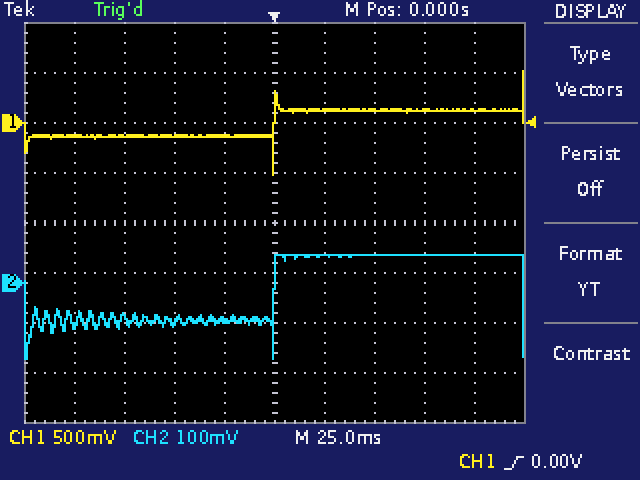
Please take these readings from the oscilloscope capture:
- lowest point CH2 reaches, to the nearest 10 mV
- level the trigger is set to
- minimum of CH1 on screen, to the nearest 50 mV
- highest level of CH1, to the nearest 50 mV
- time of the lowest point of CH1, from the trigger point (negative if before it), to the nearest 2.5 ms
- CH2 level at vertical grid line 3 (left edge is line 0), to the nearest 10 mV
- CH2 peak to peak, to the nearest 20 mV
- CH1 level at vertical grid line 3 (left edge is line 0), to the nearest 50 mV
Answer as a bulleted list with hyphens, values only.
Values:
- -150 mV
- 0.00 V
- -500 mV
- 500 mV
- 0.0 ms
- -80 mV
- 200 mV
- -150 mV
